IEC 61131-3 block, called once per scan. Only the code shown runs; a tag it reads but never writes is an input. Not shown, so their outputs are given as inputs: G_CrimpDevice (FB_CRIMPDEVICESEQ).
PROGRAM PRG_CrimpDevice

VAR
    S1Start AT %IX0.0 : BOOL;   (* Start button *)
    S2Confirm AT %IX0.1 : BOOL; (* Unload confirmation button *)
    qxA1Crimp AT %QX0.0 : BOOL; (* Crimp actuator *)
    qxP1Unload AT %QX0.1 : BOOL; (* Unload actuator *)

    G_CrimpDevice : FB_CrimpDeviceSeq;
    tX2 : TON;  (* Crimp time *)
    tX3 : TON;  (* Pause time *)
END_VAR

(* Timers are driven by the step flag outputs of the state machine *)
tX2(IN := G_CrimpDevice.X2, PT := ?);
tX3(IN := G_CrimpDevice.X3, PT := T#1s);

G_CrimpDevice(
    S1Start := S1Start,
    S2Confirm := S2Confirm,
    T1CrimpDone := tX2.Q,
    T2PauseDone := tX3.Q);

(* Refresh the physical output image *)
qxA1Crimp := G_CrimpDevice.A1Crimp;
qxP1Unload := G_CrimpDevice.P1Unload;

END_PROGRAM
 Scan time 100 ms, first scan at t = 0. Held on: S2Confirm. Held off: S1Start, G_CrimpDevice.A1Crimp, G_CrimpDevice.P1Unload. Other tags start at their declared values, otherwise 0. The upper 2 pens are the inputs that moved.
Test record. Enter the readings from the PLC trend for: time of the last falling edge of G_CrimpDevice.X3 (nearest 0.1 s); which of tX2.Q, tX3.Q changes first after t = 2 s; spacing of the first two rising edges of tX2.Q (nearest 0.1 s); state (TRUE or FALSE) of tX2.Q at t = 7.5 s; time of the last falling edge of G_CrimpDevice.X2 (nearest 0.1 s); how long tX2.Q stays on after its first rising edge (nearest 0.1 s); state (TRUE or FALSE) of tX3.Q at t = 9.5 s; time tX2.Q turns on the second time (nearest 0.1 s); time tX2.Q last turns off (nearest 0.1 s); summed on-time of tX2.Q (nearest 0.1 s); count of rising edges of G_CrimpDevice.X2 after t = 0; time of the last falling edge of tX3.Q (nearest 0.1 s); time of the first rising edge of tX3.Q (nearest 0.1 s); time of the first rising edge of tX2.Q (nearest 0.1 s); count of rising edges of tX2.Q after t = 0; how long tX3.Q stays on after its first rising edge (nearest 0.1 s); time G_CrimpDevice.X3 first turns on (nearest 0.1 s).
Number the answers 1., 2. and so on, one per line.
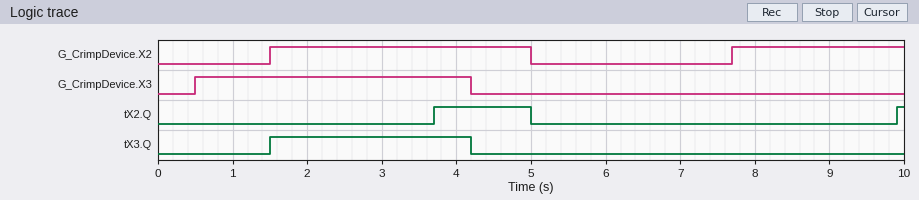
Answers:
1. 4.2 s
2. tX2.Q
3. 6.2 s
4. FALSE
5. 5.0 s
6. 1.3 s
7. FALSE
8. 9.9 s
9. 5.0 s
10. 1.4 s
11. 2
12. 4.2 s
13. 1.5 s
14. 3.7 s
15. 2
16. 2.7 s
17. 0.5 s
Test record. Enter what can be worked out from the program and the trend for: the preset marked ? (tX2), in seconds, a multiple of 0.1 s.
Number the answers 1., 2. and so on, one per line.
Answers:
1. 2.2 s
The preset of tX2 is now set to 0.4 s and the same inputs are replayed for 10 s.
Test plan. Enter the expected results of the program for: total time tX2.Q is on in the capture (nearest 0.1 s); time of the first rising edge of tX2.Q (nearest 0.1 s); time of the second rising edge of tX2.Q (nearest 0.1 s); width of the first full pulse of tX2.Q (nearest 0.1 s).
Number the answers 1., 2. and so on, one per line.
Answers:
1. 5.0 s
2. 1.9 s
3. 8.1 s
4. 3.1 s
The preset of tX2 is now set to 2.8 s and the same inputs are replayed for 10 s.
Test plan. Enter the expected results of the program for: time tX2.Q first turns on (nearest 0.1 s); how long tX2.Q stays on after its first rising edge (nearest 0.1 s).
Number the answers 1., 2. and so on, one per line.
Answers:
1. 4.3 s
2. 0.7 s
